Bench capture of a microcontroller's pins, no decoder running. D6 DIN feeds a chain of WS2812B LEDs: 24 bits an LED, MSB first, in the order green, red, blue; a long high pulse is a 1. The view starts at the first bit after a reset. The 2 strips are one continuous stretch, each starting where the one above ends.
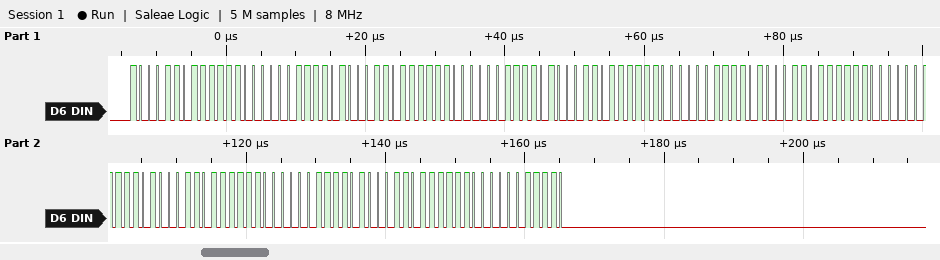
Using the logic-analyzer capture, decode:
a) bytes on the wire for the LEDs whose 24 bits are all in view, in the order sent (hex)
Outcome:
8D F8 1E 8D F8 1E 8D F8 1E 8D F8 1E 8D F8 1E 8D F8 1E
